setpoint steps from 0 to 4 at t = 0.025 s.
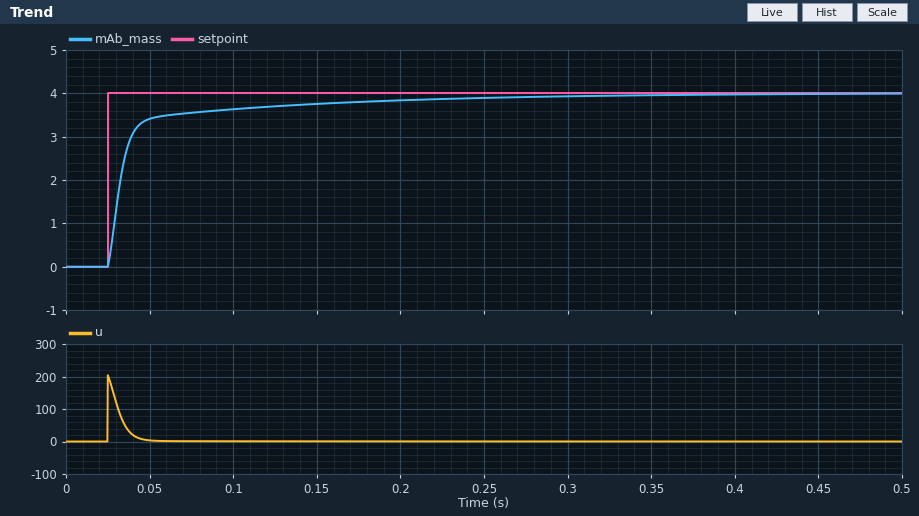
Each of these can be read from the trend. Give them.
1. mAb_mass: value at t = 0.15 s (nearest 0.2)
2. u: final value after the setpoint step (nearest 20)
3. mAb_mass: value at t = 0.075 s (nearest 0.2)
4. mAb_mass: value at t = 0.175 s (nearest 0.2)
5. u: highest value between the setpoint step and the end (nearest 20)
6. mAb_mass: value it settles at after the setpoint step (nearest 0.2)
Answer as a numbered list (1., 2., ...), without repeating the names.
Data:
1. 3.8
2. 0
3. 3.6
4. 3.8
5. 200
6. 4.0
